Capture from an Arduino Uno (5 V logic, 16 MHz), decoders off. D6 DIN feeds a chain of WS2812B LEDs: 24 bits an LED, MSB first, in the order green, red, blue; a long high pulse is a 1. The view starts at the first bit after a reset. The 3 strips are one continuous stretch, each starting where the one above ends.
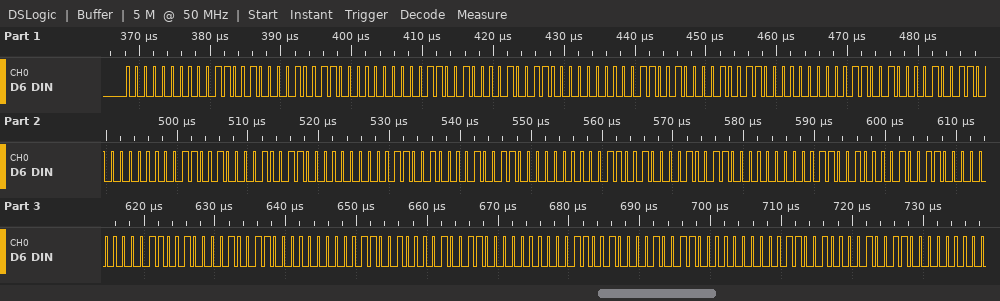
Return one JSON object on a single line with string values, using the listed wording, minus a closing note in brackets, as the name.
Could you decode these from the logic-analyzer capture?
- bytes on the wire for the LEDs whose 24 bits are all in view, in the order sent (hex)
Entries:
{"bytes on the wire for the LEDs whose 24 bits are all in view, in the order sent": "00 32 13 00 32 13 00 32 13 00 32 13 00 32 13 00 32 13 00 32 13 00 32 13 00 32 13 00 32 13 00 32 13 00 32 13"}
